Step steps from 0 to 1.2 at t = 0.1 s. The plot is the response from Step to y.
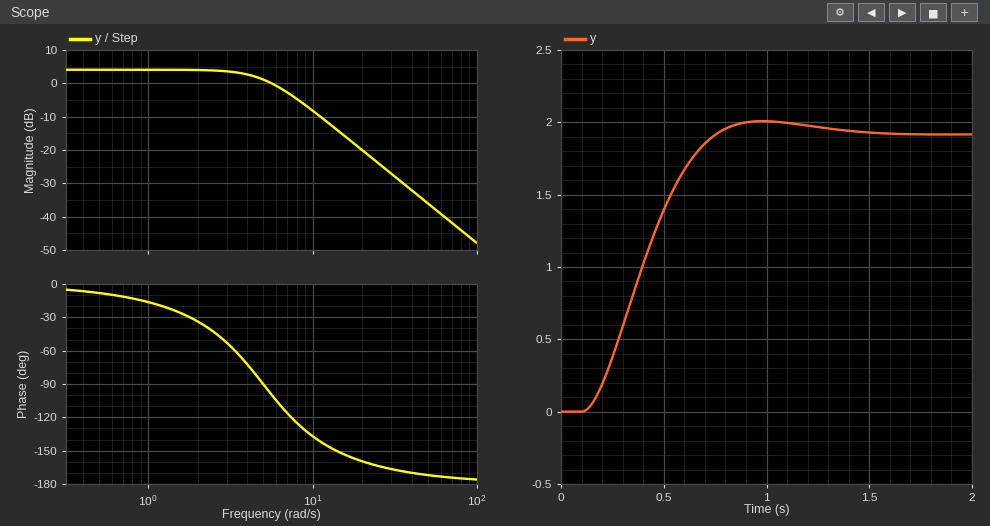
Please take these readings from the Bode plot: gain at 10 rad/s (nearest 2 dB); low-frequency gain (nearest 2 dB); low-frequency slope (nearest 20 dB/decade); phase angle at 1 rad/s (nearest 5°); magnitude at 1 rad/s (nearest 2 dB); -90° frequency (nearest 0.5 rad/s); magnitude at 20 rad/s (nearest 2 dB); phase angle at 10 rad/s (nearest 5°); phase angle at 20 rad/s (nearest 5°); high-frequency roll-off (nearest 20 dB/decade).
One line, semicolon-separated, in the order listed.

-8 dB; 4 dB; 0 dB/decade; -15°; 4 dB; 5.0 rad/s; -20 dB; -135°; -160°; -40 dB/decade
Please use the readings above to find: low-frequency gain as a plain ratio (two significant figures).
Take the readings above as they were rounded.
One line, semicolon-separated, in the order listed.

1.6
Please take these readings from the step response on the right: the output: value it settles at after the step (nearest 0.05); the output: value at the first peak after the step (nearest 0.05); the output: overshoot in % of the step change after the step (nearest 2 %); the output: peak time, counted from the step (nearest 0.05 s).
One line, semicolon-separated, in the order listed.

1.90; 2.00; 4 %; 0.90 s
